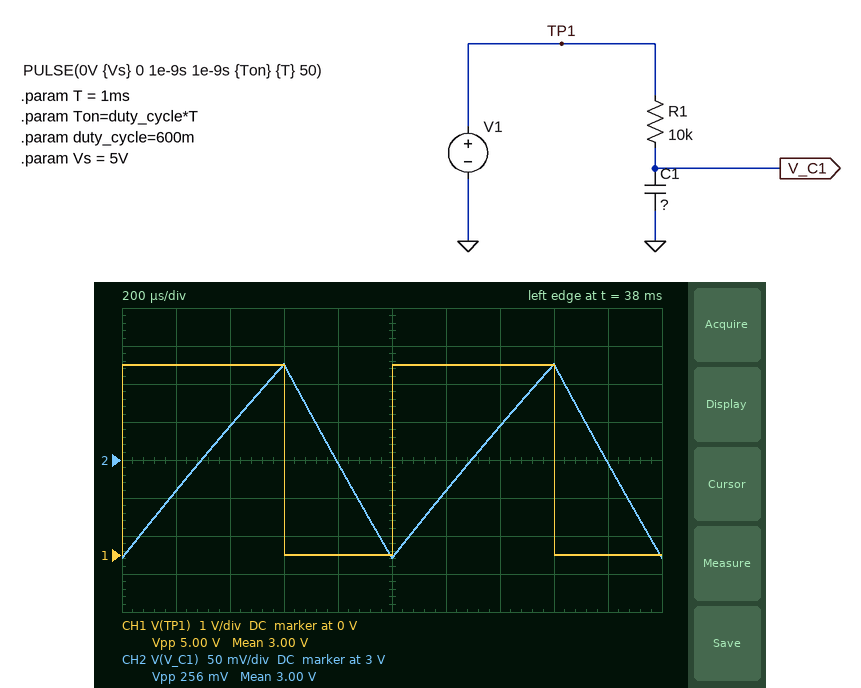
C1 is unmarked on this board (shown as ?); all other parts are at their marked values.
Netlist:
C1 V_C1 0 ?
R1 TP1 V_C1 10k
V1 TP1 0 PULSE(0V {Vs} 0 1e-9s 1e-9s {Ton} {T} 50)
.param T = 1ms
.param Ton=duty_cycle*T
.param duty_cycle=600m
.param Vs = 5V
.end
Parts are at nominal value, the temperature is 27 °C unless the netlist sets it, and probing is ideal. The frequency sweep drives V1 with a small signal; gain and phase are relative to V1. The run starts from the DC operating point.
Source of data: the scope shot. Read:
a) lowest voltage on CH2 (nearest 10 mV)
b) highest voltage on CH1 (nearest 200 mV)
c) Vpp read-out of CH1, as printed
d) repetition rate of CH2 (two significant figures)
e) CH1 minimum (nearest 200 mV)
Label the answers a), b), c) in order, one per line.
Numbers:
a) 2.87 V
b) 5.0 V
c) 5.00 V
d) 1.0 kHz
e) 0 V
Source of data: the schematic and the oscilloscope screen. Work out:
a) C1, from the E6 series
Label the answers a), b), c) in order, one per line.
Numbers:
a) 470 nF
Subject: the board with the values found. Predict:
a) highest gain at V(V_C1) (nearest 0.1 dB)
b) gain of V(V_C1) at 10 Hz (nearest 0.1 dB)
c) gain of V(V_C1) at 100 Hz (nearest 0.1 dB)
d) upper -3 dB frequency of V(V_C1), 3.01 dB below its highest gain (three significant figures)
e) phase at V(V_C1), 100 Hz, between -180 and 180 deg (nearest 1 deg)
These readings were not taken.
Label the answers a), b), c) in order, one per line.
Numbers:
a) 0 dB
b) -0.4 dB
c) -9.9 dB
d) 33.9 Hz
e) -71 deg
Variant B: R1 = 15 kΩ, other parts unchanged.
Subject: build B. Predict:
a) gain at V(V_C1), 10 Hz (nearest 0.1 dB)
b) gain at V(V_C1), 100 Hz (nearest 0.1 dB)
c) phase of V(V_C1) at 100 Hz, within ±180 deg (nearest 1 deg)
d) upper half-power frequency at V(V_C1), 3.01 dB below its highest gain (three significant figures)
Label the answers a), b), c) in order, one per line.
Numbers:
a) -0.8 dB
b) -13.1 dB
c) -77 deg
d) 22.6 Hz
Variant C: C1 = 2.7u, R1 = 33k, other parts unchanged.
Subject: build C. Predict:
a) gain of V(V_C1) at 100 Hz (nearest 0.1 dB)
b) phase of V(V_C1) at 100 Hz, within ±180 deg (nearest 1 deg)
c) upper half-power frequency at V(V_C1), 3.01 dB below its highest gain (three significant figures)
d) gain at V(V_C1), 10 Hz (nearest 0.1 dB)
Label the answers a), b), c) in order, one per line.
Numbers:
a) -35.0 dB
b) -89 deg
c) 1.79 Hz
d) -15.1 dB
